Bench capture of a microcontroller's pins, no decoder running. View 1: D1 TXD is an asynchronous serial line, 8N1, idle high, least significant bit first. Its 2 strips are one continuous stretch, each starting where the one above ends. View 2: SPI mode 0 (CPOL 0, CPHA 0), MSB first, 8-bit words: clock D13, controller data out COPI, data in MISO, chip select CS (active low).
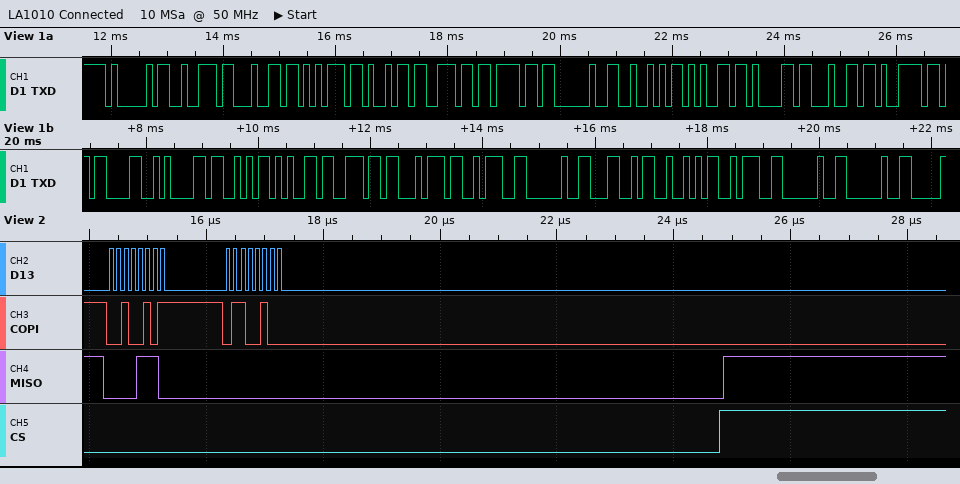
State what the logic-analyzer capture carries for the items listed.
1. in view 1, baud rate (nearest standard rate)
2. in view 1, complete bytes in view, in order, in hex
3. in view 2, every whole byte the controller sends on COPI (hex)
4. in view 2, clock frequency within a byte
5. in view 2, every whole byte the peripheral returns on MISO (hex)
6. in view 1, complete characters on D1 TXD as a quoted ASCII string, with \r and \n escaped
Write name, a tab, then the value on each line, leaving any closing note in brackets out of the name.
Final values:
in view 1, baud rate	9600 baud
in view 1, complete bytes in view, in order, in hex	41 72 64 75 69 6E 6F 20 52 65 61 64 79 0D 0A 53 65 6E 74 3A 20 4C 52 3A 20 20
in view 2, every whole byte the controller sends on COPI	25 64
in view 2, clock frequency within a byte	8 MHz
in view 2, every whole byte the peripheral returns on MISO	0E 00
in view 1, complete characters on D1 TXD as a quoted ASCII string, with \r and \n escaped	"Arduino Ready\r\nSent: LR:  "
